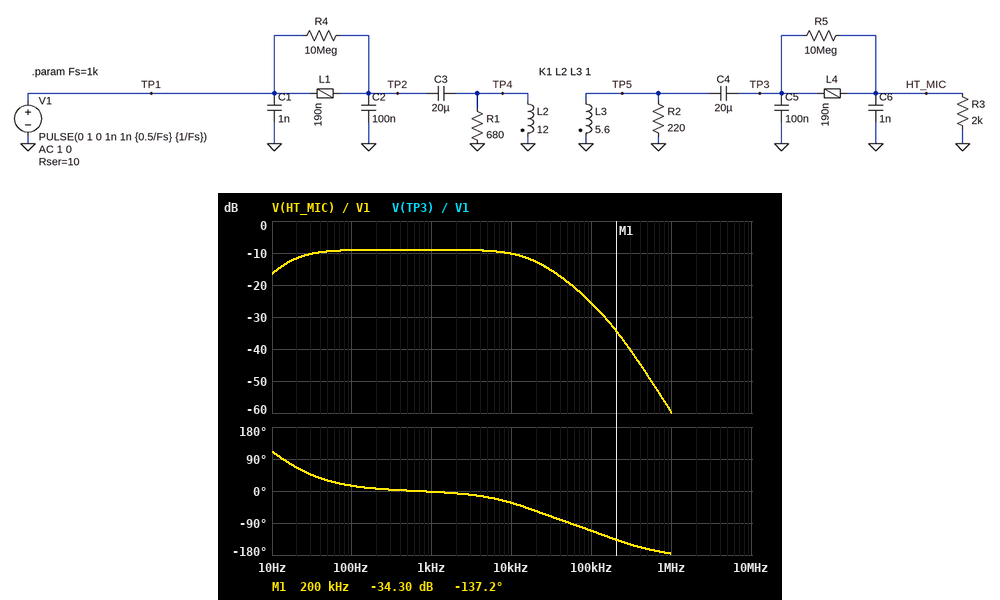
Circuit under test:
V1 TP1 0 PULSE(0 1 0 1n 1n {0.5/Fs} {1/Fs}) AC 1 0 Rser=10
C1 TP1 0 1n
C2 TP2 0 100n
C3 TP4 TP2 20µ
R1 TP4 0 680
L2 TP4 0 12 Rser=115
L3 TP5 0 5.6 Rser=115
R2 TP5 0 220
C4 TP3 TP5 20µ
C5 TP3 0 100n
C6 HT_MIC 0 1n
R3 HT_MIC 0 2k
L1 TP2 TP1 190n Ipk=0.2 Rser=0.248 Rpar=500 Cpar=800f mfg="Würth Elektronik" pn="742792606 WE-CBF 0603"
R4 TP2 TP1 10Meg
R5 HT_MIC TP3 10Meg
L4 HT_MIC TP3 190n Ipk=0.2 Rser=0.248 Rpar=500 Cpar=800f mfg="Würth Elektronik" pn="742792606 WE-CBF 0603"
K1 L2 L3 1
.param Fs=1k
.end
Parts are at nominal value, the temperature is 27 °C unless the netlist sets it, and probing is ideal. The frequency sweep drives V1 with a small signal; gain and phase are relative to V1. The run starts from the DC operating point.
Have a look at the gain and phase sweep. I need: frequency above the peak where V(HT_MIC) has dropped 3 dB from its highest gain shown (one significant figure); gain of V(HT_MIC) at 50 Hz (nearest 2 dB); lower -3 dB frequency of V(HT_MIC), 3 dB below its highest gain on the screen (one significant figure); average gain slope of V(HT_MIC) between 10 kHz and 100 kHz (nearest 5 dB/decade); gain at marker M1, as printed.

20 kHz
-10 dB
20 Hz
-15 dB/decade
-34.30 dB
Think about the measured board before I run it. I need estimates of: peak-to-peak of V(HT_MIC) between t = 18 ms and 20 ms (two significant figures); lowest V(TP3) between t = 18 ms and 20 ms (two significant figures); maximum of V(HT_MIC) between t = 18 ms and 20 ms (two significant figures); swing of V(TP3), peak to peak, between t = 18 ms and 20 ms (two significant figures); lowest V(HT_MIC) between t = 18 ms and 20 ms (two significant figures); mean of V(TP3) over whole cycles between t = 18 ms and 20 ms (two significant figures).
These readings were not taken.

370 mV
-210 mV
160 mV
370 mV
-210 mV
-27 mV
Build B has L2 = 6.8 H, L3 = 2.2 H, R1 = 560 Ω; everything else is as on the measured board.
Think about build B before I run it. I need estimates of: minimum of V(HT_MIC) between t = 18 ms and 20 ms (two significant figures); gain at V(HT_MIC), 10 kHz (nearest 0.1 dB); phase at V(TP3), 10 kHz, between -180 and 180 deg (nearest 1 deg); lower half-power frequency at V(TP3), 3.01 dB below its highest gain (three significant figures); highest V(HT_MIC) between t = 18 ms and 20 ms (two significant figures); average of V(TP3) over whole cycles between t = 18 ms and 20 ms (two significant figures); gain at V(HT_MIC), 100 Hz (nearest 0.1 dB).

-190 mV
-11.3 dB
-32 deg
17.7 Hz
130 mV
-33 mV
-10.2 dB
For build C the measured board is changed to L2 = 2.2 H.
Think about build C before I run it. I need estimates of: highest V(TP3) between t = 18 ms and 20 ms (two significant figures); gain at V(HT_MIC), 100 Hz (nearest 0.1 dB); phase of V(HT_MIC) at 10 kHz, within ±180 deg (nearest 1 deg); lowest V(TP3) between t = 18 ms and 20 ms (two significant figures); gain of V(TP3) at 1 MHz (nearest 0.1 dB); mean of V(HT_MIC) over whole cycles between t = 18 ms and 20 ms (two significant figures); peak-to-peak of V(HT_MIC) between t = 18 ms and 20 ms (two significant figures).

230 mV
-6.8 dB
-44 deg
-290 mV
-60.4 dB
-28 mV
520 mV
